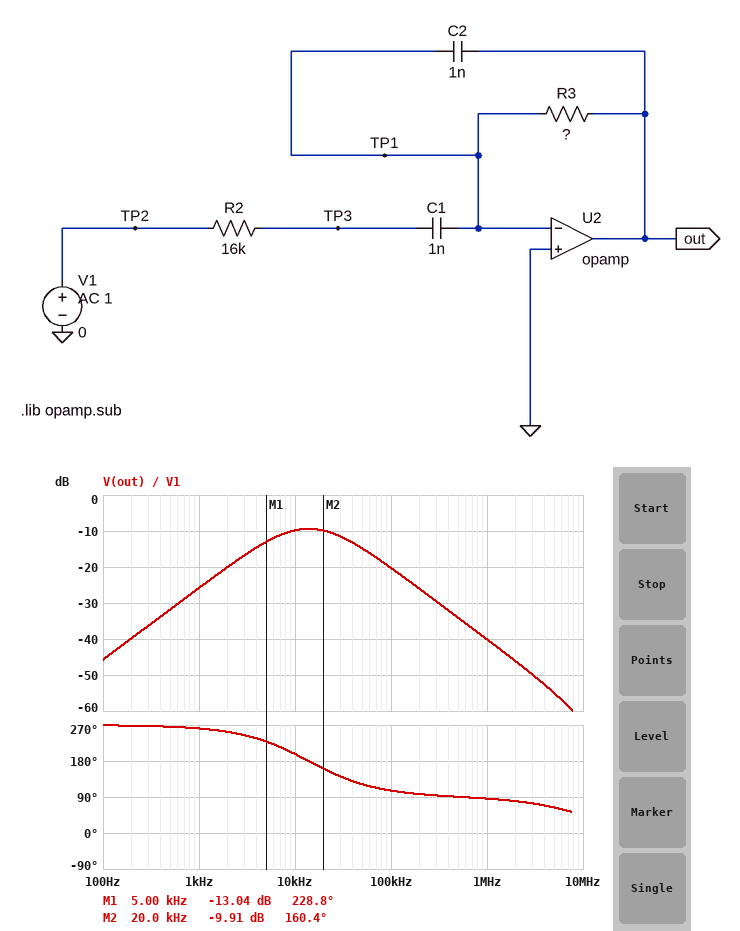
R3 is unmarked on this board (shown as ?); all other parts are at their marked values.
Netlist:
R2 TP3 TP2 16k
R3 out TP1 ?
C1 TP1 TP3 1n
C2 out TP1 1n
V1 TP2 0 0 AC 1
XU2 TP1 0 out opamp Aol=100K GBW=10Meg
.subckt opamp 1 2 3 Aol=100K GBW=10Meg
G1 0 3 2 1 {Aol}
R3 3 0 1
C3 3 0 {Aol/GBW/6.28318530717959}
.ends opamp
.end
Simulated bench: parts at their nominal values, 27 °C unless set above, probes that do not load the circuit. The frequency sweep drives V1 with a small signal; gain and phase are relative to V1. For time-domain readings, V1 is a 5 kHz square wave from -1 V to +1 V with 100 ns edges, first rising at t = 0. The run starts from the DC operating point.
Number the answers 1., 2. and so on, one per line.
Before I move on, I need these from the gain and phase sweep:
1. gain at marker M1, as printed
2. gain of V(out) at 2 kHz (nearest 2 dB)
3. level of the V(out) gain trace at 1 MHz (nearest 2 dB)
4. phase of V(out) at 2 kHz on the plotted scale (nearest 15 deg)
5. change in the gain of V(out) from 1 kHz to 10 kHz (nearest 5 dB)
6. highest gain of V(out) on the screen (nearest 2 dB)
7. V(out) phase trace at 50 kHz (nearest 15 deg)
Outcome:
1. -13.04 dB
2. -20 dB
3. -40 dB
4. 255 deg
5. 15 dB
6. -10 dB
7. 120 deg
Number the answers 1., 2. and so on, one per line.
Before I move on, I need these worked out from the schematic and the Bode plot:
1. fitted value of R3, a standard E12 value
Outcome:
1. 8.2 kΩ
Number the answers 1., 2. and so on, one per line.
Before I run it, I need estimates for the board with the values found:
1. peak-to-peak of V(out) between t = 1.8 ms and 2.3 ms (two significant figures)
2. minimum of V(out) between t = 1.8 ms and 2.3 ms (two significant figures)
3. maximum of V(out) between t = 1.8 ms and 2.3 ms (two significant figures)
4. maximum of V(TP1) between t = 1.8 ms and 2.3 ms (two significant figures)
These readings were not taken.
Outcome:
1. 1.0 V
2. -510 mV
3. 510 mV
4. 2.0 mV
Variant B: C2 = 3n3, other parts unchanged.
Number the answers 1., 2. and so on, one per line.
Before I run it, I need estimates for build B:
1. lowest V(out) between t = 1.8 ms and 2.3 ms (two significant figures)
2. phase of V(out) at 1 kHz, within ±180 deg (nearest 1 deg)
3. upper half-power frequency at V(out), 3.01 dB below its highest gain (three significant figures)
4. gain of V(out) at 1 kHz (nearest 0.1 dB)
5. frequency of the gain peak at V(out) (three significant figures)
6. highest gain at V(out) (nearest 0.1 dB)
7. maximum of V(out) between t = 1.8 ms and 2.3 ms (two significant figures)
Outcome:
1. -270 mV
2. -105 deg
3. 18.9 kHz
4. -25.9 dB
5. 7.65 kHz
6. -14.4 dB
7. 270 mV
